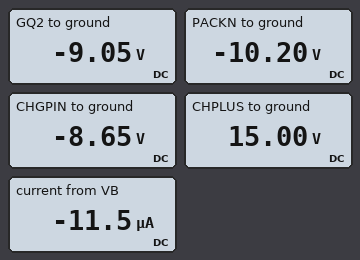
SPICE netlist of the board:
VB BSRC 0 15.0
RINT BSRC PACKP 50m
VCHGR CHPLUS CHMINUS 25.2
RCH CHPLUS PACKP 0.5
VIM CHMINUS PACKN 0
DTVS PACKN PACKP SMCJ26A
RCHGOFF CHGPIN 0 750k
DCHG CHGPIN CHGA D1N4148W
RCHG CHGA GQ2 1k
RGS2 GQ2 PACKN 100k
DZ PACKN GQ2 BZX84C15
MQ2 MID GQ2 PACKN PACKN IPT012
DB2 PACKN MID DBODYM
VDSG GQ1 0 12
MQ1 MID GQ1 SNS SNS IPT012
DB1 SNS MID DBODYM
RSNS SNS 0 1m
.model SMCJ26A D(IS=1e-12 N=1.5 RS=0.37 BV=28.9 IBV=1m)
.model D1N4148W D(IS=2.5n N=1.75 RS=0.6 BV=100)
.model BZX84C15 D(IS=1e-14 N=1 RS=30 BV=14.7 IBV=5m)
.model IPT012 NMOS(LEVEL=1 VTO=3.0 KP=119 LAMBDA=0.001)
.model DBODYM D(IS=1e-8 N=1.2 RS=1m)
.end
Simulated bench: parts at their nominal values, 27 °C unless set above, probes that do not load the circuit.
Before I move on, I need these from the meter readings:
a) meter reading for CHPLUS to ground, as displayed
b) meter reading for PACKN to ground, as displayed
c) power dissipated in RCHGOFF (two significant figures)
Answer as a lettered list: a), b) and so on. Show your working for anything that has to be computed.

a) 15.00 V
b) -10.20 V
c) (0 V - (-8.65 V))^2 / 750 kΩ = 100 µW
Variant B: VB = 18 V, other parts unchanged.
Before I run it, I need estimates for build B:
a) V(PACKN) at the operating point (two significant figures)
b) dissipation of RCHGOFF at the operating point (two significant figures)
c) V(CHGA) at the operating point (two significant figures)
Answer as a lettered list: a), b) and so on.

a) -7.2 V
b) 48 µW
c) -6.4 V
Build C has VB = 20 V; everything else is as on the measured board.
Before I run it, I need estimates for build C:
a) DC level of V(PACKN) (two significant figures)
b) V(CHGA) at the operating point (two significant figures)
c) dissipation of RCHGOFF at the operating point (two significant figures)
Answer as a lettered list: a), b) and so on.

a) -5.2 V
b) -4.6 V
c) 24 µW
